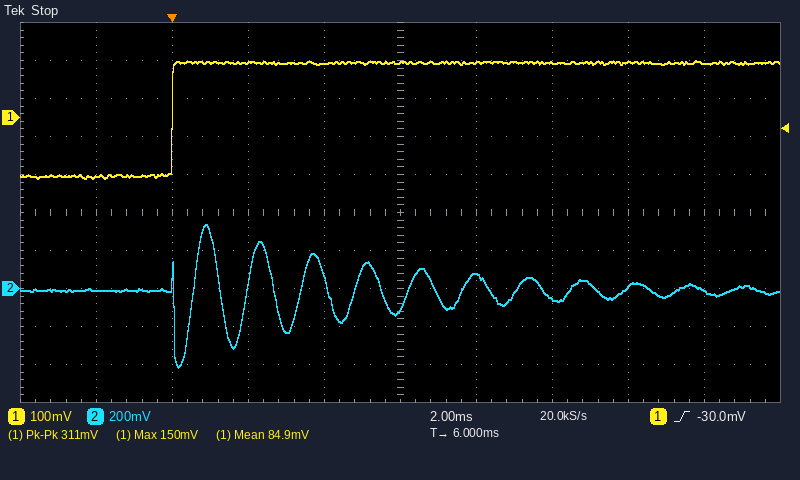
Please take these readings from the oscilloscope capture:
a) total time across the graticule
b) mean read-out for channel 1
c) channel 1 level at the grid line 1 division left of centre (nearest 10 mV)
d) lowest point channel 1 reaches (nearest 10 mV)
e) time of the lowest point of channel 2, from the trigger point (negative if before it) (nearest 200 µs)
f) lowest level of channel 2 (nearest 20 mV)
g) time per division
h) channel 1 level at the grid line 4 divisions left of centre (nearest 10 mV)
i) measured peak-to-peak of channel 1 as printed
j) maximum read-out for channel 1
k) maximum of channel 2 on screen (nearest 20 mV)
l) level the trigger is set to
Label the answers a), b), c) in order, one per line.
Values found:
a) 20 ms
b) 84.9 mV
c) 140 mV
d) -160 mV
e) +200 µs
f) -420 mV
g) 2 ms
h) -160 mV
i) 311 mV
j) 150 mV
k) 340 mV
l) -30.0 mV
